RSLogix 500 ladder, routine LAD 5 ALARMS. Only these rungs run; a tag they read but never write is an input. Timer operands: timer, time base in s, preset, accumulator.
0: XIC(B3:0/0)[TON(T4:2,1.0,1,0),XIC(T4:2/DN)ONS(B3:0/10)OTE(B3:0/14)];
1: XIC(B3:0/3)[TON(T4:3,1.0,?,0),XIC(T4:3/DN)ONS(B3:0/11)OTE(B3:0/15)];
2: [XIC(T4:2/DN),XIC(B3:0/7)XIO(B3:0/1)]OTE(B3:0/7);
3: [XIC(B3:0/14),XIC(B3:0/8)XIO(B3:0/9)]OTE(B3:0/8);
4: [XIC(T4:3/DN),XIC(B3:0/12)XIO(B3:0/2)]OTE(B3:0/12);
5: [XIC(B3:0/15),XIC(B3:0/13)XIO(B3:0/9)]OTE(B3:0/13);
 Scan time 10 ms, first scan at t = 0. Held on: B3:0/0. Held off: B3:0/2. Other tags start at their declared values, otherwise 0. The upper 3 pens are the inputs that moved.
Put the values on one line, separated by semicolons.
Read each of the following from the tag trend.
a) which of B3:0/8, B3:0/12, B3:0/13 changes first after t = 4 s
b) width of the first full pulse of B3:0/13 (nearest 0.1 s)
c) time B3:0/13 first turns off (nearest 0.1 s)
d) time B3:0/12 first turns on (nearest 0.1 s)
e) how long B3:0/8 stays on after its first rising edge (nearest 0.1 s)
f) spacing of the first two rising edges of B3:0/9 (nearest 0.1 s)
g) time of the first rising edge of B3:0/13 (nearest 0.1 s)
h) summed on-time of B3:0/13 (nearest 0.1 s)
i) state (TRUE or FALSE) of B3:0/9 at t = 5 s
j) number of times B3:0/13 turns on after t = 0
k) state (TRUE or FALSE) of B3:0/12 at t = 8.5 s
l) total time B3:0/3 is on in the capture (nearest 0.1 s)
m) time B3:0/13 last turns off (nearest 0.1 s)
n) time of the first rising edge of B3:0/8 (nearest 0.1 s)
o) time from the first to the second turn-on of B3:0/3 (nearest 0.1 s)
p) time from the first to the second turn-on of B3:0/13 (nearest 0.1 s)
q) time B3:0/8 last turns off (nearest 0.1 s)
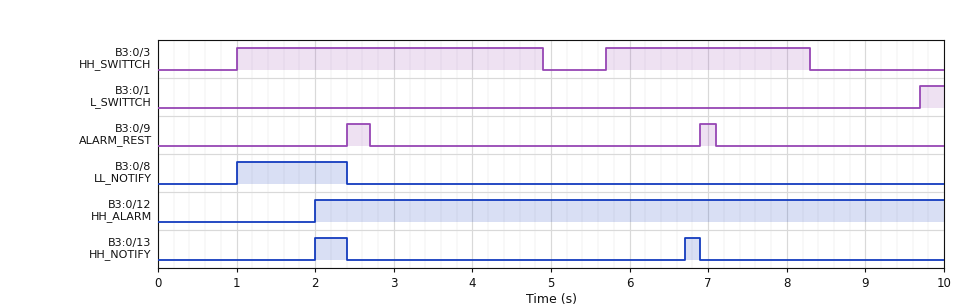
B3:0/13; 0.4 s; 2.4 s; 2.0 s; 1.4 s; 4.5 s; 2.0 s; 0.6 s; FALSE; 2; TRUE; 6.5 s; 6.9 s; 1.0 s; 4.7 s; 4.7 s; 2.4 s
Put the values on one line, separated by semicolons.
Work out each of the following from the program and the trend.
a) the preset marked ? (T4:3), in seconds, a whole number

1 s
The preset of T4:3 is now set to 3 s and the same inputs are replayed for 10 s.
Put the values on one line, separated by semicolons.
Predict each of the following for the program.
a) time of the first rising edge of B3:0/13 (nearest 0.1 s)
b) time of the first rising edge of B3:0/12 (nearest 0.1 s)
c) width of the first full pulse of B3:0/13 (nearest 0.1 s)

4.0 s; 4.0 s; 2.9 s
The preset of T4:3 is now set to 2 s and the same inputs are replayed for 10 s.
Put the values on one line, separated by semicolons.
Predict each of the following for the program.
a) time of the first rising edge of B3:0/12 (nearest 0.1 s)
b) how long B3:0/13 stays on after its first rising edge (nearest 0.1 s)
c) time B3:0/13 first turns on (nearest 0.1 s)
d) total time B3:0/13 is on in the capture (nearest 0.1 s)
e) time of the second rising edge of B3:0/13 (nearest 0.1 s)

3.0 s; 3.9 s; 3.0 s; 6.2 s; 7.7 s
